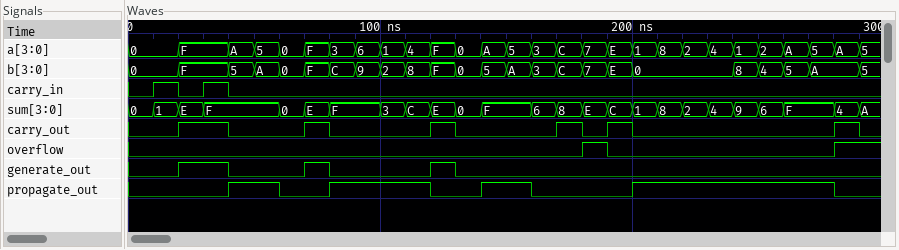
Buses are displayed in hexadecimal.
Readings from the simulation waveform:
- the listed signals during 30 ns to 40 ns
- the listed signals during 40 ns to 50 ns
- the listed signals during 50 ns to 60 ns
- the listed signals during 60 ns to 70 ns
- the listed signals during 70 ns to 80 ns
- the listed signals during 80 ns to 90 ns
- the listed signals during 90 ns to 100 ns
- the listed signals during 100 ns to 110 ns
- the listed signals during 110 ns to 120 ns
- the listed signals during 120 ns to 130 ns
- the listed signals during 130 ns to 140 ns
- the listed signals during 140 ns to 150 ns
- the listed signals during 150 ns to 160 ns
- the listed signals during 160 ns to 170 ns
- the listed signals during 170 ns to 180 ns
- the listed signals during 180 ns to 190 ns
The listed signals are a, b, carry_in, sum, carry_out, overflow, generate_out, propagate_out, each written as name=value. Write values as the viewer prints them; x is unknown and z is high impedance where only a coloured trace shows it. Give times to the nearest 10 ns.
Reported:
a=F, b=F, carry_in=1, sum=F, carry_out=1, overflow=0, generate_out=1, propagate_out=0
a=A, b=5, carry_in=0, sum=F, carry_out=0, overflow=0, generate_out=0, propagate_out=1
a=5, b=A, carry_in=0, sum=F, carry_out=0, overflow=0, generate_out=0, propagate_out=1
a=0, b=0, carry_in=0, sum=0, carry_out=0, overflow=0, generate_out=0, propagate_out=0
a=F, b=F, carry_in=0, sum=E, carry_out=1, overflow=0, generate_out=1, propagate_out=0
a=3, b=C, carry_in=0, sum=F, carry_out=0, overflow=0, generate_out=0, propagate_out=1
a=6, b=9, carry_in=0, sum=F, carry_out=0, overflow=0, generate_out=0, propagate_out=1
a=1, b=2, carry_in=0, sum=3, carry_out=0, overflow=0, generate_out=0, propagate_out=1
a=4, b=8, carry_in=0, sum=C, carry_out=0, overflow=0, generate_out=0, propagate_out=1
a=F, b=F, carry_in=0, sum=E, carry_out=1, overflow=0, generate_out=1, propagate_out=0
a=0, b=0, carry_in=0, sum=0, carry_out=0, overflow=0, generate_out=0, propagate_out=0
a=A, b=5, carry_in=0, sum=F, carry_out=0, overflow=0, generate_out=0, propagate_out=1
a=5, b=A, carry_in=0, sum=F, carry_out=0, overflow=0, generate_out=0, propagate_out=1
a=3, b=3, carry_in=0, sum=6, carry_out=0, overflow=0, generate_out=0, propagate_out=0
a=C, b=C, carry_in=0, sum=8, carry_out=1, overflow=0, generate_out=0, propagate_out=0
a=7, b=7, carry_in=0, sum=E, carry_out=0, overflow=1, generate_out=0, propagate_out=0
